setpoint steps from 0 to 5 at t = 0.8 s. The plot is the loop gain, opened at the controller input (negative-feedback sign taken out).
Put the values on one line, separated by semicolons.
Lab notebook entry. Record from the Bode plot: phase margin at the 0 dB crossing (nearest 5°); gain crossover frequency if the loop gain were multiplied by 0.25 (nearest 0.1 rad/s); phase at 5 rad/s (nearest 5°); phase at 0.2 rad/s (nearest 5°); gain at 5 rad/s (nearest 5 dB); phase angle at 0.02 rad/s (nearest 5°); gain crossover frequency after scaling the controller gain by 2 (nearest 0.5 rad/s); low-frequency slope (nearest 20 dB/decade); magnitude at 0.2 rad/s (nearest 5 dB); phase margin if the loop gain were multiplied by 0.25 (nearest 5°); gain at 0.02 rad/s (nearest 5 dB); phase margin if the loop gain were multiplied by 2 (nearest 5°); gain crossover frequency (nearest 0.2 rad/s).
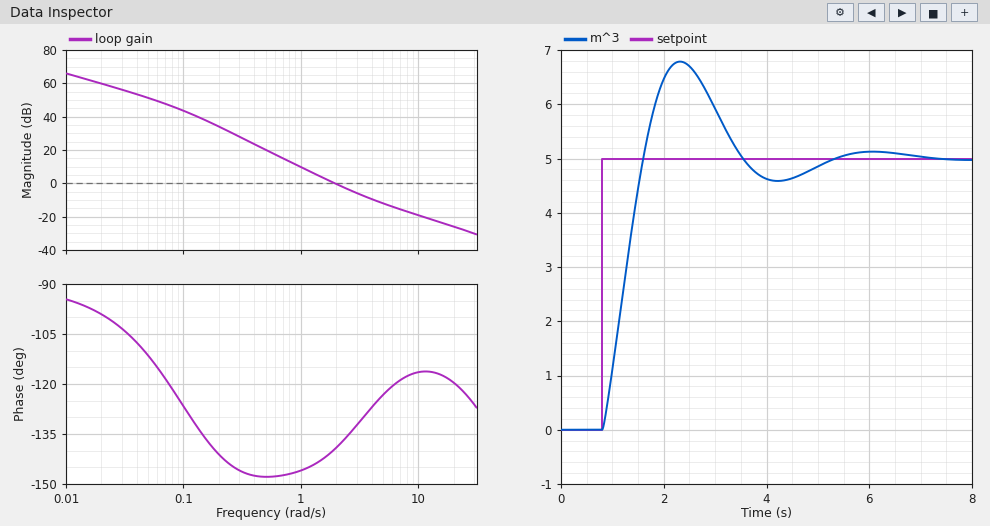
40°; 0.9 rad/s; -125°; -140°; -10 dB; -100°; 3.0 rad/s; -20 dB/decade; 35 dB; 35°; 60 dB; 50°; 2.0 rad/s
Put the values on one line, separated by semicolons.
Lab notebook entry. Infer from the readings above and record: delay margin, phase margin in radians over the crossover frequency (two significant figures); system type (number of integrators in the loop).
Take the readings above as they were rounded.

0.35 s; 1
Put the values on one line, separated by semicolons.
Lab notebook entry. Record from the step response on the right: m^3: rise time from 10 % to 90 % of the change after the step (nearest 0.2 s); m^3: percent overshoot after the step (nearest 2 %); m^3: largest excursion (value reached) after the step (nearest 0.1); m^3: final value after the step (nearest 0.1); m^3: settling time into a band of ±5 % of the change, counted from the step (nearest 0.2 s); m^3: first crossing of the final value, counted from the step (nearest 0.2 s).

0.6 s; 36 %; 6.8; 5.0; 4.0 s; 0.8 s
